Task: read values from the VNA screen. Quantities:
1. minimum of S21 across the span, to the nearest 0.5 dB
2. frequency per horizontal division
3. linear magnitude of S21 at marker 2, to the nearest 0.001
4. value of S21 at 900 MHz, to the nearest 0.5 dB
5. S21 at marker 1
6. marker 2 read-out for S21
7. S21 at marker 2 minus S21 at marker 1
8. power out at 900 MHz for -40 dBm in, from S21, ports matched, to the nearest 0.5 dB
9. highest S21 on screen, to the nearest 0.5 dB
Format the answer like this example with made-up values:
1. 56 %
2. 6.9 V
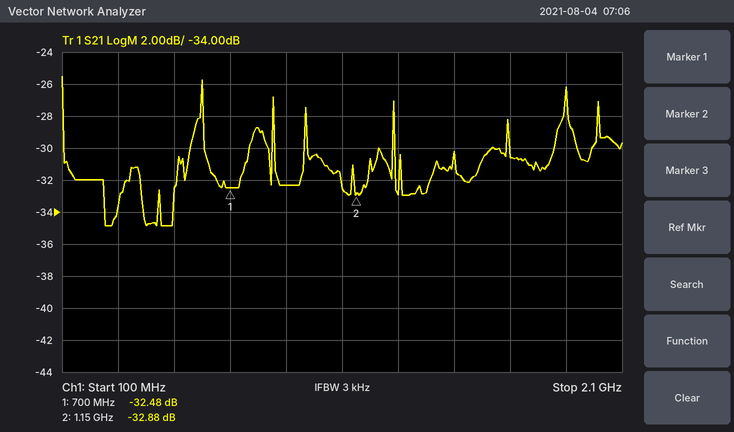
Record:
1. -35.0 dB
2. 200 MHz
3. 0.023
4. -32.5 dB
5. -32.48 dB
6. -32.88 dB
7. -0.40 dB
8. -72.5 dBm
9. -25.5 dB
